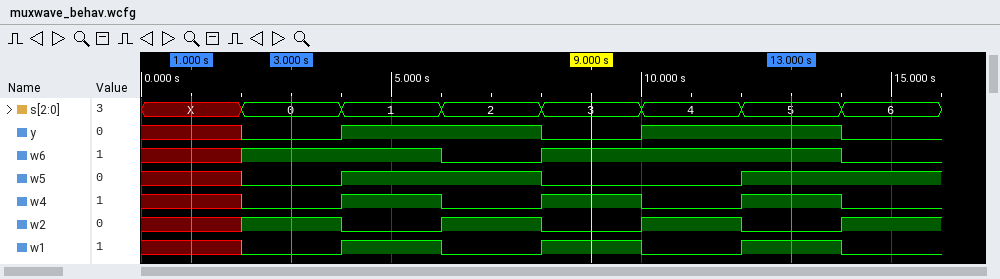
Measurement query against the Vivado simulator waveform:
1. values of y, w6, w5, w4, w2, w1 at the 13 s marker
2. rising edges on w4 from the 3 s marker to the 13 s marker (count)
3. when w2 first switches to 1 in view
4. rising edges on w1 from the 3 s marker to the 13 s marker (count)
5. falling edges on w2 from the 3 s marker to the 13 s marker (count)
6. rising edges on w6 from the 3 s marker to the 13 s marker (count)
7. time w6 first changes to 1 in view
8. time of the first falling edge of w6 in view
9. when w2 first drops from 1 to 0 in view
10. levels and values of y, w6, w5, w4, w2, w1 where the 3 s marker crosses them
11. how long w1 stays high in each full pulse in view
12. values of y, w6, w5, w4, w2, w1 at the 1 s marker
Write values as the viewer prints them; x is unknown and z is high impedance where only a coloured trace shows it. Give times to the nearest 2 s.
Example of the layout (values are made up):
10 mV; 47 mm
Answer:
y=1, w6=1, w5=1, w4=1, w2=0, w1=1; 3; 2 s; 3; 3; 1; 2 s; 6 s; 4 s; y=0, w6=1, w5=0, w4=0, w2=1, w1=0; 2 s, 2 s, 2 s; y=x, w6=x, w5=x, w4=x, w2=x, w1=x
